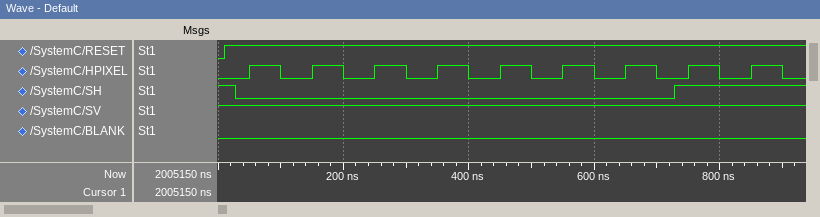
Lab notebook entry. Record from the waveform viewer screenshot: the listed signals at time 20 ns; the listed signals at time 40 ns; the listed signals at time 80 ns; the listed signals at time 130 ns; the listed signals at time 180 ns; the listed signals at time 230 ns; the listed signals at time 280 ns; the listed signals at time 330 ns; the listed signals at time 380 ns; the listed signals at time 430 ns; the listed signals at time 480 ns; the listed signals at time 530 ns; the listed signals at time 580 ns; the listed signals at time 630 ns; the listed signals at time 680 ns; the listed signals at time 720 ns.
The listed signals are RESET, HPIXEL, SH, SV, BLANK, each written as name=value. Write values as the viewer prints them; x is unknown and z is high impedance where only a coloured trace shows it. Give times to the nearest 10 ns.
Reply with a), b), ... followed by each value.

a) RESET=1, HPIXEL=0, SH=1, SV=1, BLANK=0
b) RESET=1, HPIXEL=0, SH=0, SV=1, BLANK=0
c) RESET=1, HPIXEL=1, SH=0, SV=1, BLANK=0
d) RESET=1, HPIXEL=0, SH=0, SV=1, BLANK=0
e) RESET=1, HPIXEL=1, SH=0, SV=1, BLANK=0
f) RESET=1, HPIXEL=0, SH=0, SV=1, BLANK=0
g) RESET=1, HPIXEL=1, SH=0, SV=1, BLANK=0
h) RESET=1, HPIXEL=0, SH=0, SV=1, BLANK=0
i) RESET=1, HPIXEL=1, SH=0, SV=1, BLANK=0
j) RESET=1, HPIXEL=0, SH=0, SV=1, BLANK=0
k) RESET=1, HPIXEL=1, SH=0, SV=1, BLANK=0
l) RESET=1, HPIXEL=0, SH=0, SV=1, BLANK=0
m) RESET=1, HPIXEL=1, SH=0, SV=1, BLANK=0
n) RESET=1, HPIXEL=0, SH=0, SV=1, BLANK=0
o) RESET=1, HPIXEL=1, SH=0, SV=1, BLANK=0
p) RESET=1, HPIXEL=0, SH=0, SV=1, BLANK=0
